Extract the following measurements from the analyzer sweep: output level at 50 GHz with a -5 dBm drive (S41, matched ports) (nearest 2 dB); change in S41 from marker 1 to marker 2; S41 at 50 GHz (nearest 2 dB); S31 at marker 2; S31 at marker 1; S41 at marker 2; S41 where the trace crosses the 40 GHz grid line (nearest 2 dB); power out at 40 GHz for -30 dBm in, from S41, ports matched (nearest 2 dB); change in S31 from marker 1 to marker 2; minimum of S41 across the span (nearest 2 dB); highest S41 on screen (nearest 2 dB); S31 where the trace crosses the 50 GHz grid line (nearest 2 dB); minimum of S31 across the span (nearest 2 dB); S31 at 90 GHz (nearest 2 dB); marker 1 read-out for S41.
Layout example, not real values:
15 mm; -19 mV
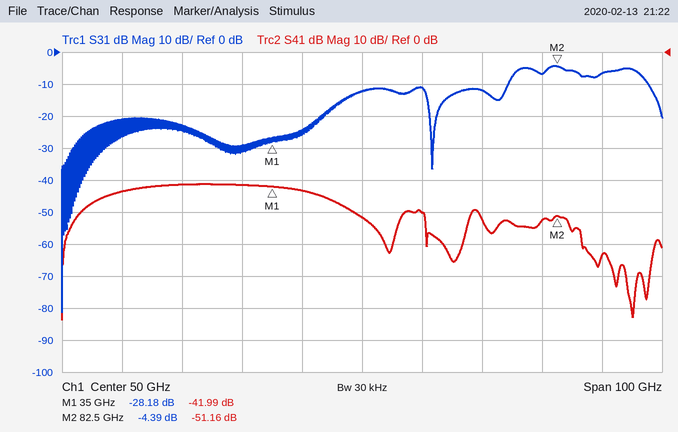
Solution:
-56 dBm; -9.17 dB; -52 dB; -4.39 dB; -28.18 dB; -51.16 dB; -44 dB; -74 dBm; 23.79 dB; -84 dB; -42 dB; -12 dB; -82 dB; -6 dB; -41.99 dB
